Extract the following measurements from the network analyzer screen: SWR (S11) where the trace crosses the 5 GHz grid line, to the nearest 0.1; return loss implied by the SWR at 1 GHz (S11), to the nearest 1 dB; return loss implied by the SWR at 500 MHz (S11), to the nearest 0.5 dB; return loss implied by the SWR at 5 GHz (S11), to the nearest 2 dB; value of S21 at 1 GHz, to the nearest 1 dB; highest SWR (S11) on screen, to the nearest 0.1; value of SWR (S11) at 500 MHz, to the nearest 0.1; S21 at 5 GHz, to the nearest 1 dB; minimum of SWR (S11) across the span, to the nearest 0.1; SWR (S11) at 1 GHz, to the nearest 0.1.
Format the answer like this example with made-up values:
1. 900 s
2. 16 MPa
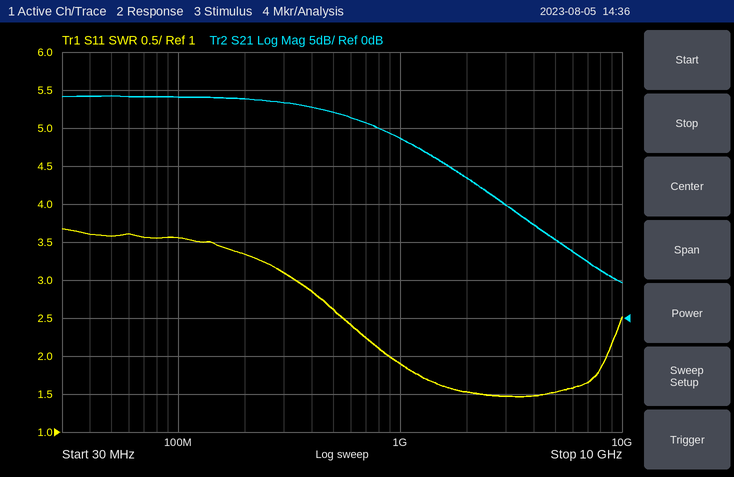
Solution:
1. 1.5
2. 10 dB
3. 7.0 dB
4. 14 dB
5. 24 dB
6. 3.7
7. 2.6
8. 10 dB
9. 1.5
10. 1.9
